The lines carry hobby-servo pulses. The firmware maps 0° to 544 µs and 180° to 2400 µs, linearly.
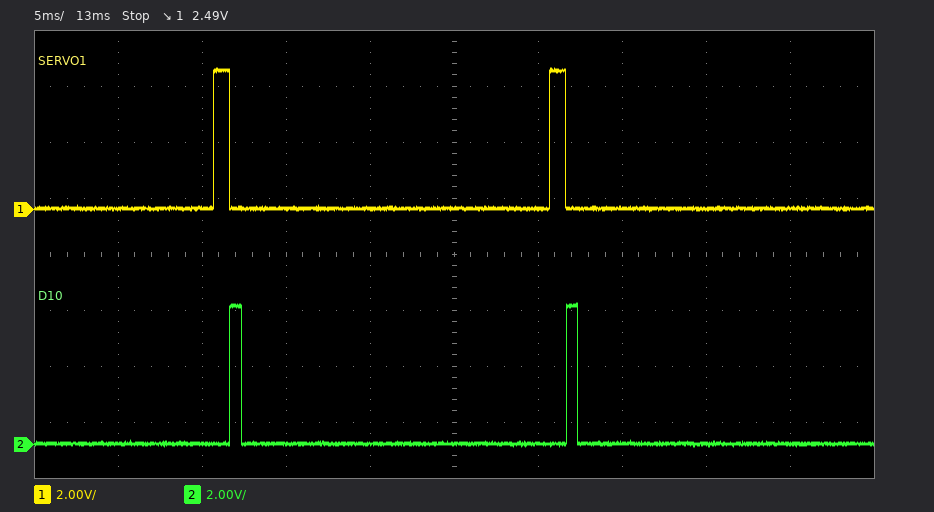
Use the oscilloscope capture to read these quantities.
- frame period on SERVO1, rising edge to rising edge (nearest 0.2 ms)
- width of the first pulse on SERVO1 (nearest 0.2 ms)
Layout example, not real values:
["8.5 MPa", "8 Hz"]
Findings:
["20.0 ms", "1.0 ms"]
